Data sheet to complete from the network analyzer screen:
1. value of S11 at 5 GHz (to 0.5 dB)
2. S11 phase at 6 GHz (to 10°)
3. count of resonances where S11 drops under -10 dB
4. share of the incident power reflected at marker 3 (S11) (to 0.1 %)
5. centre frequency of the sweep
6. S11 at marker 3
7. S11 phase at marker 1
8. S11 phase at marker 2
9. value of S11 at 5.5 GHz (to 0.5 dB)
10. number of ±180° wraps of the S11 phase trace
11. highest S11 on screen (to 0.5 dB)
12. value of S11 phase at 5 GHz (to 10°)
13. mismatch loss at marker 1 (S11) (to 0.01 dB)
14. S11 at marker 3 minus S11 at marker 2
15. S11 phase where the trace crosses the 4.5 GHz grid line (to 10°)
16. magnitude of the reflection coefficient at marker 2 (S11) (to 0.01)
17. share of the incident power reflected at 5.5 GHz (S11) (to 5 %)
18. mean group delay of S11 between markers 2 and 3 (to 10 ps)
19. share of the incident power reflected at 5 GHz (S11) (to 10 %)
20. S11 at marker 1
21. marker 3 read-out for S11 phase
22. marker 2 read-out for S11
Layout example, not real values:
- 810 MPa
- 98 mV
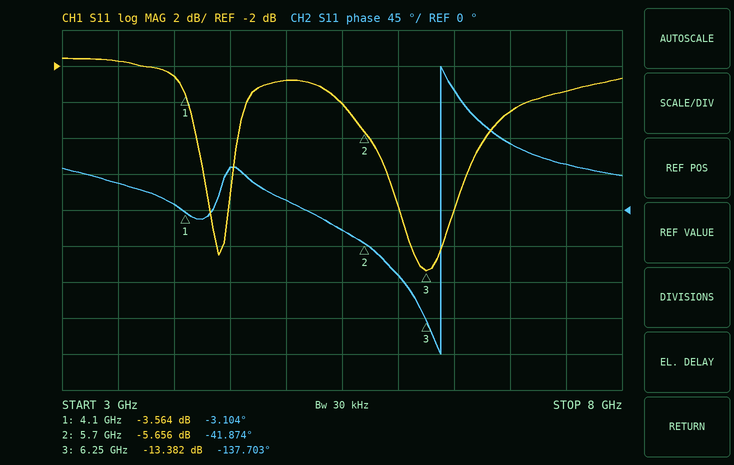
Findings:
- -3.0 dB
- -80°
- 2
- 4.6 %
- 5.5 GHz
- -13.382 dB
- -3.104°
- -41.874°
- -4.0 dB
- 1
- -1.5 dB
- 10°
- 2.52 dB
- -7.726 dB
- 50°
- 0.52
- 40 %
- 480 ps
- 50 %
- -3.564 dB
- -137.703°
- -5.656 dB
